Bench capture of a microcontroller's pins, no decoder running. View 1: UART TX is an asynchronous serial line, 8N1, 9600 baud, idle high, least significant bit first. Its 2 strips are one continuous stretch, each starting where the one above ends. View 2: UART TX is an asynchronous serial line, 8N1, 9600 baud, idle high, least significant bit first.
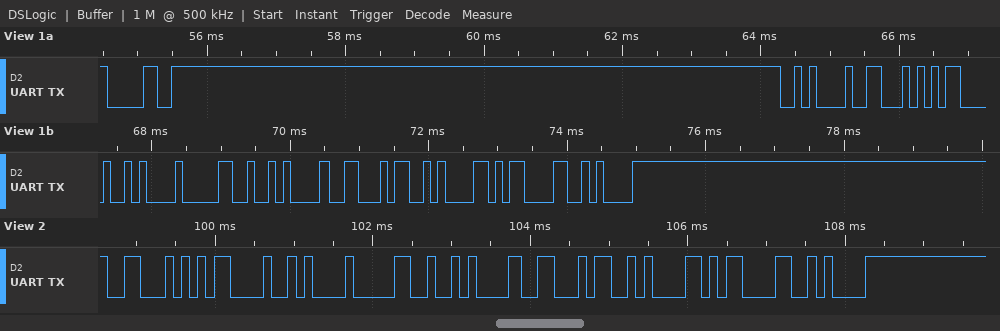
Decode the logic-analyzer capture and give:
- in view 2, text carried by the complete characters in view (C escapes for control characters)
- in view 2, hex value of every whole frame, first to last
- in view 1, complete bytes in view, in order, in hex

"F\r\n0\nF\n\r\n"
46 0D 0A 30 0A 46 0A 0D 0A
30 0A 46 0D 0A 30 0A 46 0A 0D 0A
